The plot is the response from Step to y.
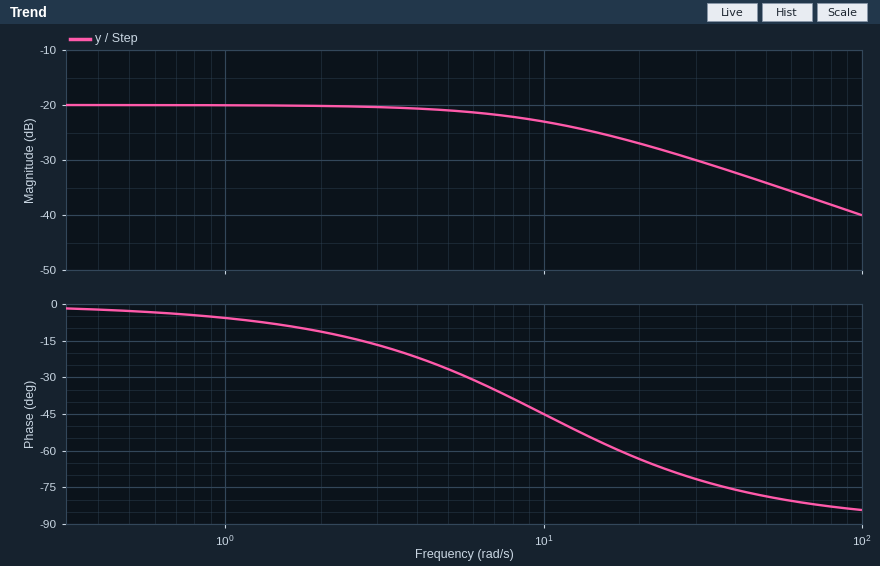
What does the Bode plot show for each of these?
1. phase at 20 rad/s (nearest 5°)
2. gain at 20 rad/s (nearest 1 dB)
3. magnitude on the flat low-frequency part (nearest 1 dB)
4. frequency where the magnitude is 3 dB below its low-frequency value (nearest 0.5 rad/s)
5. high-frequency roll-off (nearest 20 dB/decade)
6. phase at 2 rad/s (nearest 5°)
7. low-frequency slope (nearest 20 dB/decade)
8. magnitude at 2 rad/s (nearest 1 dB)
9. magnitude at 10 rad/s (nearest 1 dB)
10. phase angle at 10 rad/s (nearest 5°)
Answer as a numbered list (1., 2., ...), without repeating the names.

1. -65°
2. -27 dB
3. -20 dB
4. 10.0 rad/s
5. -20 dB/decade
6. -10°
7. 0 dB/decade
8. -20 dB
9. -23 dB
10. -45°
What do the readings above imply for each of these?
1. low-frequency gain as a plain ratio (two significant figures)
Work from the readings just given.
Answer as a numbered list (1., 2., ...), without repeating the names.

1. 0.10
